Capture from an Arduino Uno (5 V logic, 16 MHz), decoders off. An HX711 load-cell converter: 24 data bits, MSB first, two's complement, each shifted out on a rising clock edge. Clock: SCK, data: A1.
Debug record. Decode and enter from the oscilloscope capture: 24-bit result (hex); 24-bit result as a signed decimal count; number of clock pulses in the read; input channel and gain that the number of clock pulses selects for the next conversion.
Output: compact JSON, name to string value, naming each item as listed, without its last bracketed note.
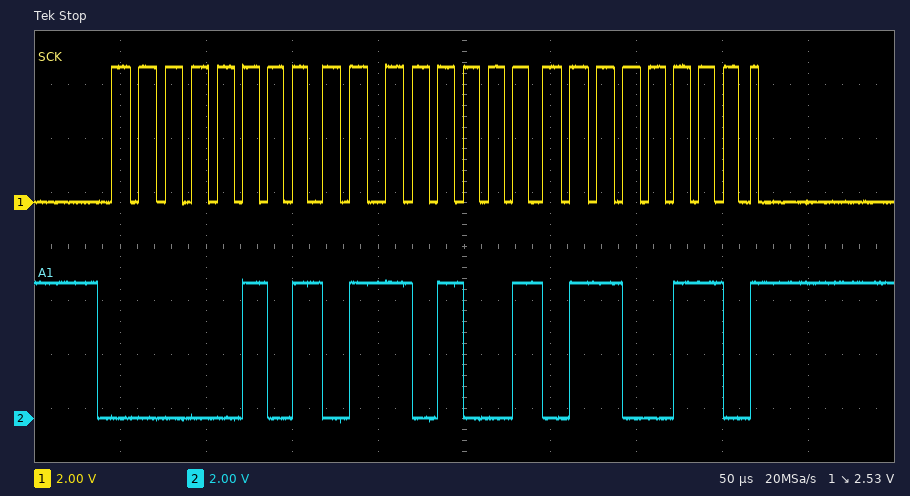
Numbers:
{"24-bit result": "0x056966", "24-bit result as a signed decimal count": "354662", "number of clock pulses in the read": "25", "input channel and gain that the number of clock pulses selects for the next conversion": "channel A, gain 128"}
